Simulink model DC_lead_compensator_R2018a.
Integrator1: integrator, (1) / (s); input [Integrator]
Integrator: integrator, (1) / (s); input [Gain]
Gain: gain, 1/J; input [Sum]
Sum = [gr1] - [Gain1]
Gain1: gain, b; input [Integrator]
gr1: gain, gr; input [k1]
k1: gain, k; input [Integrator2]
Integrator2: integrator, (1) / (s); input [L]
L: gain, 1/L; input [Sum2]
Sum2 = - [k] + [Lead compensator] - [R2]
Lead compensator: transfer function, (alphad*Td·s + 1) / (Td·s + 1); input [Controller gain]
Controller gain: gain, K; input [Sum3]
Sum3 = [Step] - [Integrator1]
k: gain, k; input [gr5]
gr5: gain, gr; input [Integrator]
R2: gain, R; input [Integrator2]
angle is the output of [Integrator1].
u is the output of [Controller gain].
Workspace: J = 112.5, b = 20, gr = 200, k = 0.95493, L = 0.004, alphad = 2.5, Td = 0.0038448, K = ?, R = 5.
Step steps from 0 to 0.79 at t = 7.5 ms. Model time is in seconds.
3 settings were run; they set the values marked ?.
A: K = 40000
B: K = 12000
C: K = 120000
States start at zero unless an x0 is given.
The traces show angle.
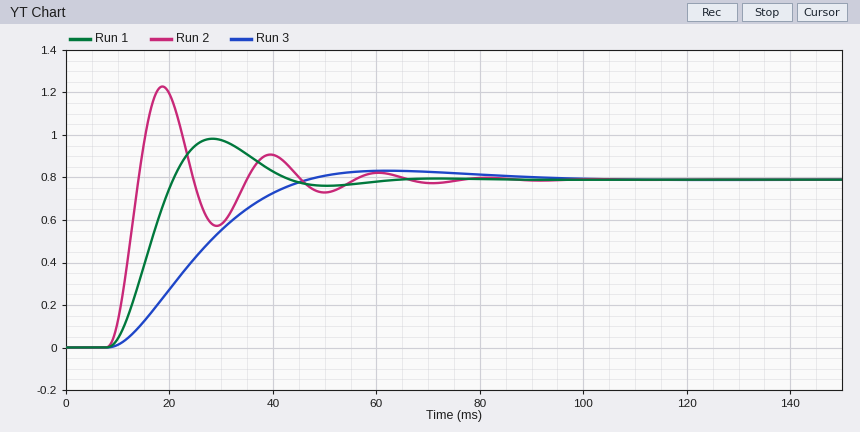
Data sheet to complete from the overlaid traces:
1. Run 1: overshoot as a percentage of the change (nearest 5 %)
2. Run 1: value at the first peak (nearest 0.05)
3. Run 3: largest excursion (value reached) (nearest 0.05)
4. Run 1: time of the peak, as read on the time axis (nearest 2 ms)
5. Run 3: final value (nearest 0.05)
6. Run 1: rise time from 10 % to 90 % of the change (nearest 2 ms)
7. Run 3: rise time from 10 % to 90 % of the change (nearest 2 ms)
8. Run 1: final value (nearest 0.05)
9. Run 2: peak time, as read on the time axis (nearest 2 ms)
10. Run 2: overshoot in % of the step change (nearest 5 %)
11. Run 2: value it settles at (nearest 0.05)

25 %
1.00
0.85
28 ms
0.80
8 ms
26 ms
0.80
18 ms
55 %
0.80
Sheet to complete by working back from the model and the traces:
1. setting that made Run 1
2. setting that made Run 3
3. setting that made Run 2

A
B
C
